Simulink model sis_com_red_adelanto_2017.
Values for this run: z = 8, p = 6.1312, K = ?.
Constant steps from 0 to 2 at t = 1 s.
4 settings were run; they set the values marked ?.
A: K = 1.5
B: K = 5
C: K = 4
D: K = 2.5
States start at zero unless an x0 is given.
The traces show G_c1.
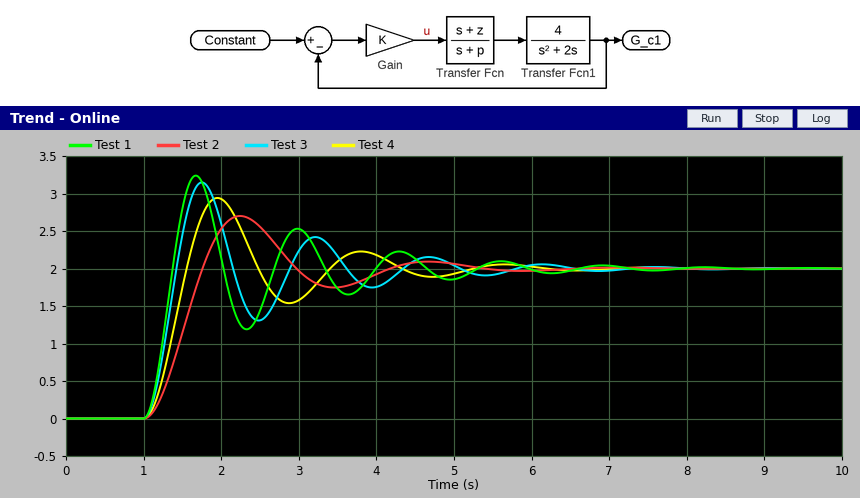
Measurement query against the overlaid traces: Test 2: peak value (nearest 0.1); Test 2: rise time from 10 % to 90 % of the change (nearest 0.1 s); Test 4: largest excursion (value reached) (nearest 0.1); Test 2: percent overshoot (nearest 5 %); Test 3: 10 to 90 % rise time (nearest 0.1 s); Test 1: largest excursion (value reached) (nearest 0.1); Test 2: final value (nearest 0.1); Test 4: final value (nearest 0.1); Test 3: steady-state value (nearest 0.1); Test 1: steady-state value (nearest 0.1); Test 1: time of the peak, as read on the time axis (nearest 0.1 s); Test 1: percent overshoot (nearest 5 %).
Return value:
2.7
0.5 s
2.9
35 %
0.3 s
3.2
2.0
2.0
2.0
2.0
1.7 s
60 %
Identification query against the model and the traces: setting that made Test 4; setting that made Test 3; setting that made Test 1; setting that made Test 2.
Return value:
D
C
B
A
